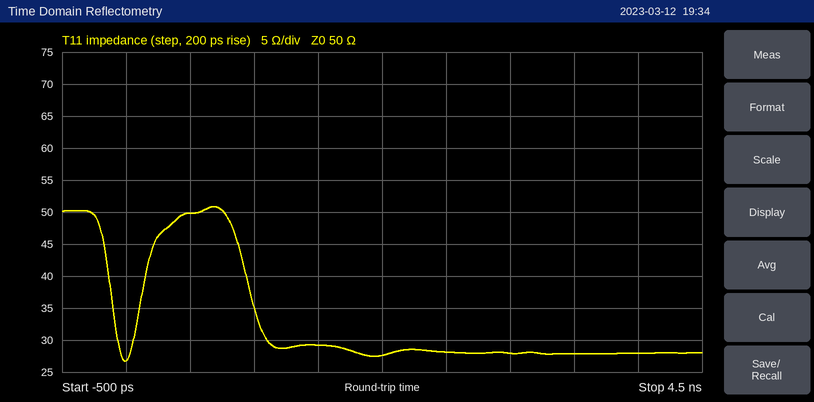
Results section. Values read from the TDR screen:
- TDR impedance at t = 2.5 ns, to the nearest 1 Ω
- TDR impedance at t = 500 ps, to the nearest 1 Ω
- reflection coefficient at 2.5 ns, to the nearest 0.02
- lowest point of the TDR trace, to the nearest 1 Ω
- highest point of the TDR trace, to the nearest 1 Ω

28 Ω
50 Ω
-0.28
27 Ω
51 Ω
